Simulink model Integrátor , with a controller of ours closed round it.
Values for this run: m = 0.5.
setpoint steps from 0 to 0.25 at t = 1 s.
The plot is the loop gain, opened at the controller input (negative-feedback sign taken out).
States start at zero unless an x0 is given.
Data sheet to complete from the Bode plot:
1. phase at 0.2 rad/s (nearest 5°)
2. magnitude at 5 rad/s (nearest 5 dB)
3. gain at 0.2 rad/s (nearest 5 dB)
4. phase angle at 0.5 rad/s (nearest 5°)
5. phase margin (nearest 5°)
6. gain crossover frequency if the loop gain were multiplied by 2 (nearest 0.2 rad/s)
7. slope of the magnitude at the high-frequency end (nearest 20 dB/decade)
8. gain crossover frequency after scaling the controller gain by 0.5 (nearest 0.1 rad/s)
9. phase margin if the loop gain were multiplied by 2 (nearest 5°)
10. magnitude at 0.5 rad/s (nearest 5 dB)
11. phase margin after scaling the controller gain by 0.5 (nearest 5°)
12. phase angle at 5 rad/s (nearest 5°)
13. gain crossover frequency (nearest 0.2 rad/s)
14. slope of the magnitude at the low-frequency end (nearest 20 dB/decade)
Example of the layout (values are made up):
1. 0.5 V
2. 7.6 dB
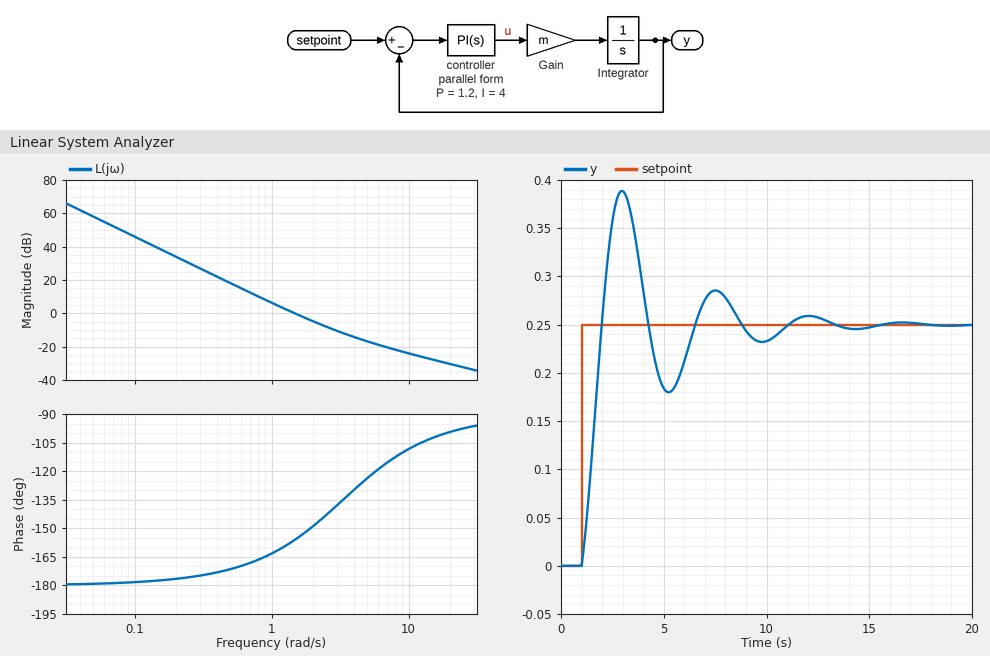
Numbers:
1. -175°
2. -15 dB
3. 35 dB
4. -170°
5. 25°
6. 2.2 rad/s
7. -20 dB/decade
8. 1.0 rad/s
9. 35°
10. 20 dB
11. 15°
12. -125°
13. 1.4 rad/s
14. -40 dB/decade
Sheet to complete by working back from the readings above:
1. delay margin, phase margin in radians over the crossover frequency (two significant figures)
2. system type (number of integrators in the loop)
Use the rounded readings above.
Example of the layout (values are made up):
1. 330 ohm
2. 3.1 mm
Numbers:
1. 0.31 s
2. 2
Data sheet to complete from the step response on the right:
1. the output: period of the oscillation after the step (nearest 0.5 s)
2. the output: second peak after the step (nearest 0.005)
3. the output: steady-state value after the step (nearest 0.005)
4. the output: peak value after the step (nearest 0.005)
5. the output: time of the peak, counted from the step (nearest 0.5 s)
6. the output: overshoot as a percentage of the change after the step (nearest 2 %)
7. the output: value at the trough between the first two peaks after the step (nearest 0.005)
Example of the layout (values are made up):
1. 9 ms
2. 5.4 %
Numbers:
1. 4.5 s
2. 0.285
3. 0.250
4. 0.390
5. 2.0 s
6. 56 %
7. 0.180
